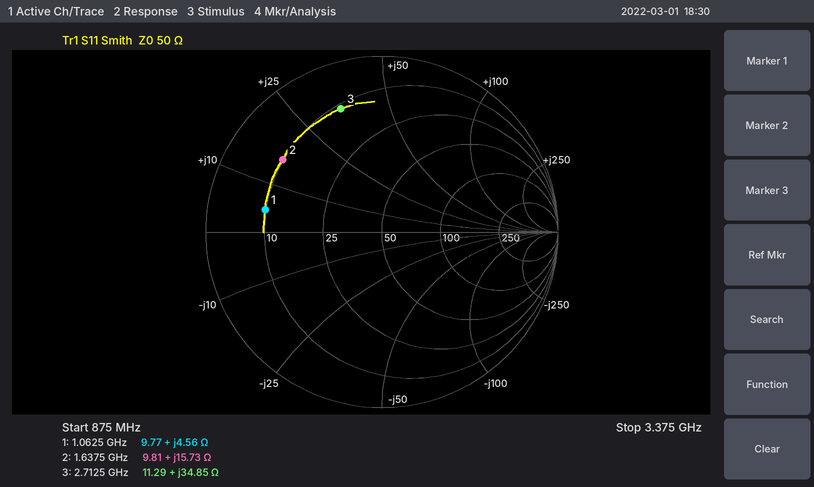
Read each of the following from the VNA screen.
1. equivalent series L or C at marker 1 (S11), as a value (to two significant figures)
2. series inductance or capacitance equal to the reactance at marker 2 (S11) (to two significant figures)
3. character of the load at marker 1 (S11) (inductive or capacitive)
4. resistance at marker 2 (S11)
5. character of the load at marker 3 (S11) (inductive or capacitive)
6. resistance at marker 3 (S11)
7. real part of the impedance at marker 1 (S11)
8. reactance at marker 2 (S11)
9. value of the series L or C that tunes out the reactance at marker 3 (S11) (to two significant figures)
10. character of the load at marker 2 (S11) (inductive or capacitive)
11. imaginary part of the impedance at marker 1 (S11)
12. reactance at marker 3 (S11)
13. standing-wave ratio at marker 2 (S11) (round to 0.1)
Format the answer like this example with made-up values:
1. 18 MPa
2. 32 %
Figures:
1. 680 pH
2. 1.5 nH
3. inductive
4. 9.81 Ω
5. inductive
6. 11.29 Ω
7. 9.77 Ω
8. +15.73 Ω
9. 1.7 pF
10. inductive
11. +4.56 Ω
12. +34.85 Ω
13. 5.6
